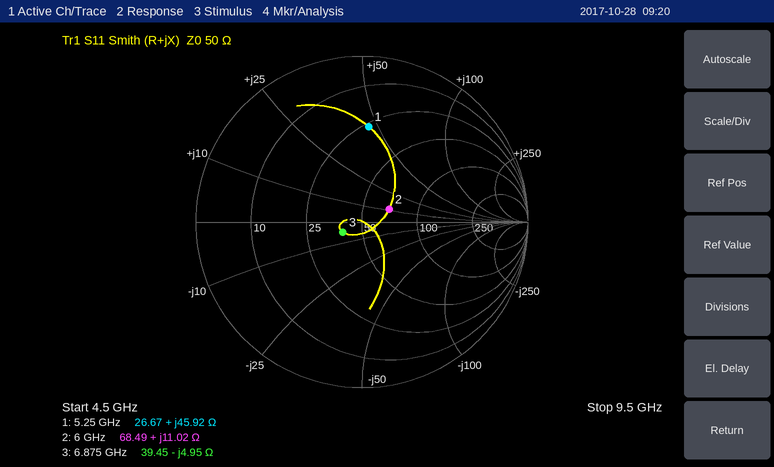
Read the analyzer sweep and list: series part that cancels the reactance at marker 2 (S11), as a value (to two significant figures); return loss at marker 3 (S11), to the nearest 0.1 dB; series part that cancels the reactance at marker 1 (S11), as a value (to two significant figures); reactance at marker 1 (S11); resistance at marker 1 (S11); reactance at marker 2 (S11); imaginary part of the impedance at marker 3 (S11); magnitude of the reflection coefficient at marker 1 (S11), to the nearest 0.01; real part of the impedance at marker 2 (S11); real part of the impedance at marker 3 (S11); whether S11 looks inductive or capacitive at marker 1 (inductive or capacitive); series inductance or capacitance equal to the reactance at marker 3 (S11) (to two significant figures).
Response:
2.4 pF
17.7 dB
660 fF
+45.92 Ω
26.67 Ω
+11.02 Ω
-4.95 Ω
0.58
68.49 Ω
39.45 Ω
inductive
4.7 pF
